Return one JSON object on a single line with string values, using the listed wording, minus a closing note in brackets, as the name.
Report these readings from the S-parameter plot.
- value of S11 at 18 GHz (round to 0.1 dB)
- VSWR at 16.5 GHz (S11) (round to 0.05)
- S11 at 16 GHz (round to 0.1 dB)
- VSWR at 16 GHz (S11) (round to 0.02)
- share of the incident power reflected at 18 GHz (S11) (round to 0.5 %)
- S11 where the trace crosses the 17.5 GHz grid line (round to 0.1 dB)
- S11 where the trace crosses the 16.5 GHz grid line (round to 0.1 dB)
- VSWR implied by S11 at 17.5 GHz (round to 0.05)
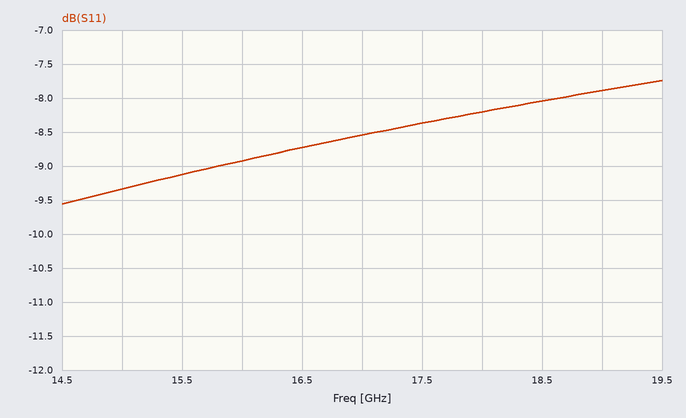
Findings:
{"value of S11 at 18 GHz": "-8.2 dB", "VSWR at 16.5 GHz (S11)": "2.15", "S11 at 16 GHz": "-8.9 dB", "VSWR at 16 GHz (S11)": "2.12", "share of the incident power reflected at 18 GHz (S11)": "15.0 %", "S11 where the trace crosses the 17.5 GHz grid line": "-8.4 dB", "S11 where the trace crosses the 16.5 GHz grid line": "-8.7 dB", "VSWR implied by S11 at 17.5 GHz": "2.25"}
